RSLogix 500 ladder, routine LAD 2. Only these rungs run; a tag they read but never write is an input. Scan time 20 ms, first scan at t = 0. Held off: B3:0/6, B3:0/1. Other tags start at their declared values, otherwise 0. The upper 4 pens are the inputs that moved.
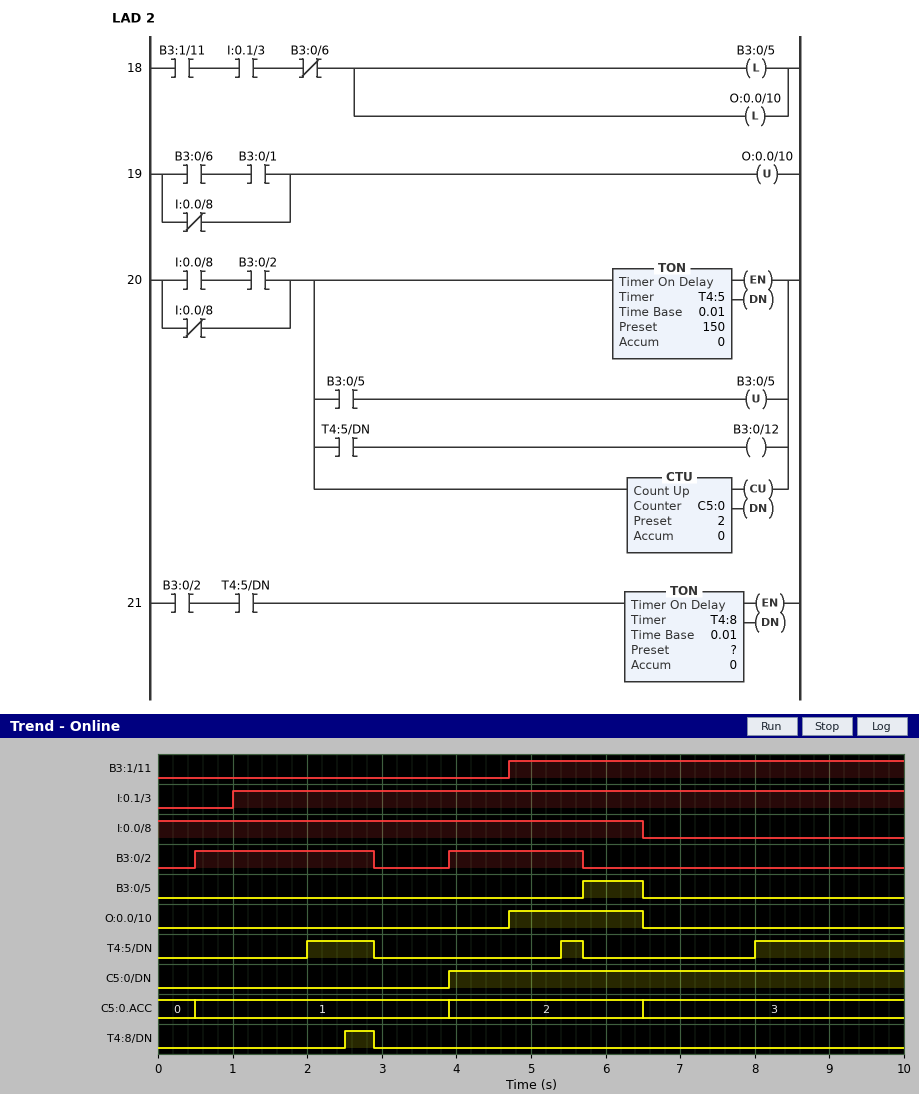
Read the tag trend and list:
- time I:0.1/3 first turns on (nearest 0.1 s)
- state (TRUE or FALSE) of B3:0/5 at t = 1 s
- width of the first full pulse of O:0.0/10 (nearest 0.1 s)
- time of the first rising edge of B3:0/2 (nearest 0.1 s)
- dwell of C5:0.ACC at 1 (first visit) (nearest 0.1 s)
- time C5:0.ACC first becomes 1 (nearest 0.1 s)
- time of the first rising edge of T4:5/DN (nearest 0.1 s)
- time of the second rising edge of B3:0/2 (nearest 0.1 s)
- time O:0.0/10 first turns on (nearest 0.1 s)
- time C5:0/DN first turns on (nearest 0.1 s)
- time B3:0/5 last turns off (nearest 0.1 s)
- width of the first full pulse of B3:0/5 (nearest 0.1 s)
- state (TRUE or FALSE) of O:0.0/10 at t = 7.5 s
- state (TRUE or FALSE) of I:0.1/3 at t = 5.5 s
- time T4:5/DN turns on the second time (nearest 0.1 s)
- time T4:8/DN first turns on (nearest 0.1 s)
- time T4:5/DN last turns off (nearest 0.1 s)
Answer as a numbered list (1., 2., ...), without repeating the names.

1. 1.0 s
2. FALSE
3. 1.8 s
4. 0.5 s
5. 3.4 s
6. 0.5 s
7. 2.0 s
8. 3.9 s
9. 4.7 s
10. 3.9 s
11. 6.5 s
12. 0.8 s
13. FALSE
14. TRUE
15. 5.4 s
16. 2.5 s
17. 5.7 s
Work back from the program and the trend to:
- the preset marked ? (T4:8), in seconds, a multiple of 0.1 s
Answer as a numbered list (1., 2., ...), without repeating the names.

1. 0.5 s
